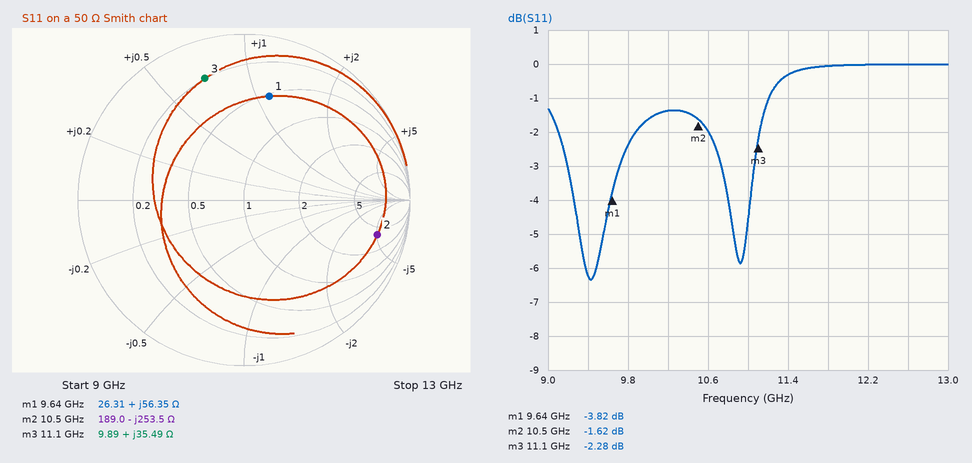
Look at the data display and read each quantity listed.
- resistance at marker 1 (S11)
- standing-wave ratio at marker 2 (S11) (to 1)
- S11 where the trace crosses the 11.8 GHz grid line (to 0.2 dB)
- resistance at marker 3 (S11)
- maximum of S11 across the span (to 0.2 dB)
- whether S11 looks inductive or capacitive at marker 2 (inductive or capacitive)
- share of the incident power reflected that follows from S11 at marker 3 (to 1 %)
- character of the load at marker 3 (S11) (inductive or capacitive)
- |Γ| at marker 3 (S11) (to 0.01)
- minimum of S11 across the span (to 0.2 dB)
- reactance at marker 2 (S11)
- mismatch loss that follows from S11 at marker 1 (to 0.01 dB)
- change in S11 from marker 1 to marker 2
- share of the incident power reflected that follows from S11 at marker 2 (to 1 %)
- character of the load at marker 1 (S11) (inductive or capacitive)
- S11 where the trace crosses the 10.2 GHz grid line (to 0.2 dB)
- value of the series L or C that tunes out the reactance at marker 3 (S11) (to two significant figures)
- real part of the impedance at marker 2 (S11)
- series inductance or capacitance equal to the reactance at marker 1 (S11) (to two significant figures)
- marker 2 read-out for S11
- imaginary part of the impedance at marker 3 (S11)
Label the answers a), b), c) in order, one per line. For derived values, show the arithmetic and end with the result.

a) 26.31 Ω
b) 11
c) 0.0 dB
d) 9.89 Ω
e) 0.0 dB
f) capacitive
g) 10^(-2.28/10) ≈ 59 %
h) inductive
i) 0.77
j) -6.4 dB
k) -253.5 Ω
l) −10 log10(1 − 10^(-3.82/10)) ≈ 2.33 dB
m) -1.62 − (-3.82) = 2.20 dB
n) 10^(-1.62/10) ≈ 69 %
o) inductive
p) -1.4 dB
q) C = 1/(2π × 11.1 GHz × 35.49 Ω) ≈ 404 fF, so 400 fF to two significant figures
r) 189.0 Ω
s) L = 56.35 Ω/(2π × 9.64 GHz) ≈ 930 pH
t) -1.62 dB
u) +35.49 Ω
